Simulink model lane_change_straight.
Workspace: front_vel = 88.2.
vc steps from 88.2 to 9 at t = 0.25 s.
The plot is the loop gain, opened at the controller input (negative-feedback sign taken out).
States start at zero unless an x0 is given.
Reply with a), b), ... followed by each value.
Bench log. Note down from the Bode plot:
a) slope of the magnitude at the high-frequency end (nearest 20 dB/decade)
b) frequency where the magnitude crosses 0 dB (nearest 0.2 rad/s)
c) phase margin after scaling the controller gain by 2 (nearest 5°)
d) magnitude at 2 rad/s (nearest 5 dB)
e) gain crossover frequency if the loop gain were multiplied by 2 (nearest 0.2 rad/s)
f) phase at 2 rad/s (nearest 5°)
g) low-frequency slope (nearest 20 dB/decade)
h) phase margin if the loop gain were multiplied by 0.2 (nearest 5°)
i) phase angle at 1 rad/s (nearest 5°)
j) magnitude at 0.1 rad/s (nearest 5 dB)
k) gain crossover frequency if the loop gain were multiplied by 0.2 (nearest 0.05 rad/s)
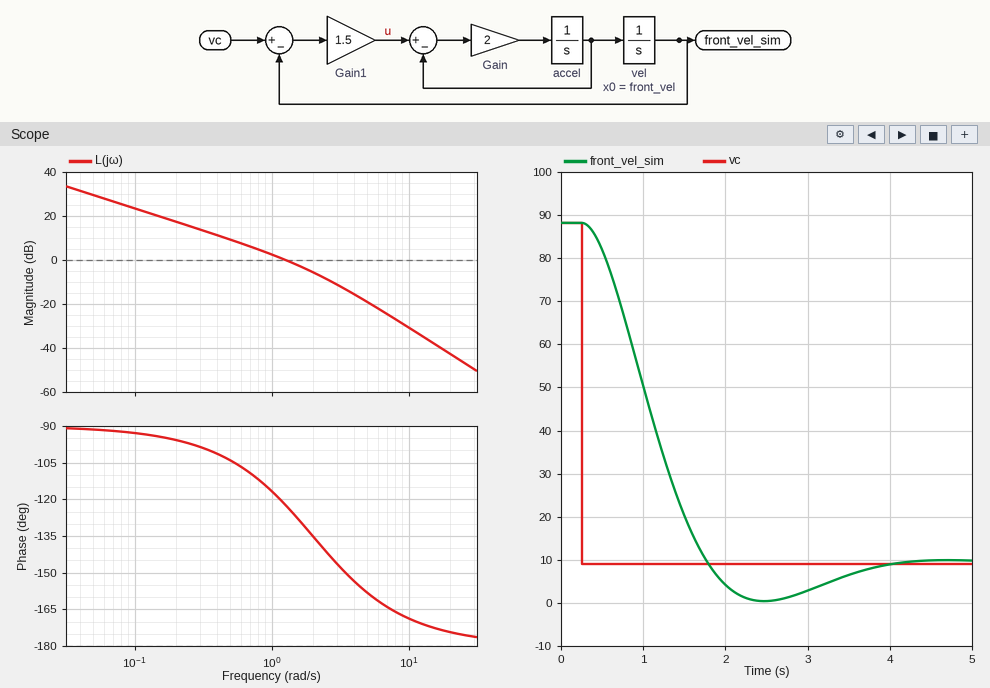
a) -40 dB/decade
b) 1.2 rad/s
c) 45°
d) -5 dB
e) 2.0 rad/s
f) -135°
g) -20 dB/decade
h) 80°
i) -115°
j) 25 dB
k) 0.30 rad/s
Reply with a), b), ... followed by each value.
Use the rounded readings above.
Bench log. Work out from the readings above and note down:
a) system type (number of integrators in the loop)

a) 1
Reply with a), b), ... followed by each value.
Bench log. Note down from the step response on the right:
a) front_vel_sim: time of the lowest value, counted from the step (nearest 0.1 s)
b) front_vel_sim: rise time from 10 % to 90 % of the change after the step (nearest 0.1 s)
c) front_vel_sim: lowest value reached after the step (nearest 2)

a) 2.2 s
b) 1.0 s
c) 0
